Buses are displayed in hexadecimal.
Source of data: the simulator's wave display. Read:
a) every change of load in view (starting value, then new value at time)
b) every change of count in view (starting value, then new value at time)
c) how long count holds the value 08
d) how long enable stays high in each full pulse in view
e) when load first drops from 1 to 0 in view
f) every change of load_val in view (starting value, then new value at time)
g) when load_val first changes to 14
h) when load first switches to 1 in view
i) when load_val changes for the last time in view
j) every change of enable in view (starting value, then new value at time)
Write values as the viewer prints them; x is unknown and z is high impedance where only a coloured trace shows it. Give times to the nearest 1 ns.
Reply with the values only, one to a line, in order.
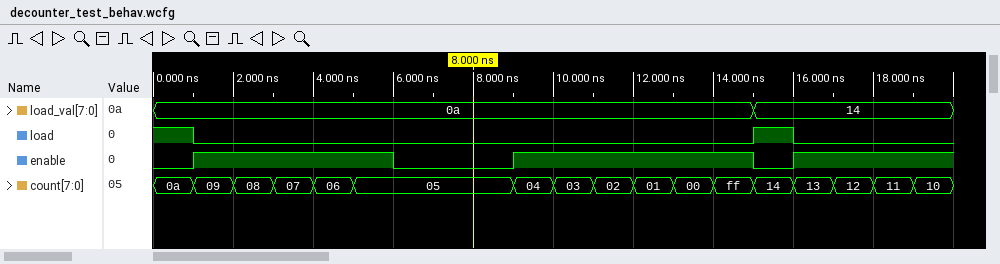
1, 0 at 1 ns, 1 at 15 ns, 0 at 16 ns
0a, 09 at 1 ns, 08 at 2 ns, 07 at 3 ns, 06 at 4 ns, 05 at 5 ns, 04 at 9 ns, 03 at 10 ns, 02 at 11 ns, 01 at 12 ns, 00 at 13 ns, ff at 14 ns, 14 at 15 ns, 13 at 16 ns, 12 at 17 ns, 11 at 18 ns, 10 at 19 ns
1 ns
5 ns, 6 ns
1 ns
0a, 14 at 15 ns
15 ns
15 ns
15 ns
0, 1 at 1 ns, 0 at 6 ns, 1 at 9 ns, 0 at 15 ns, 1 at 16 ns
